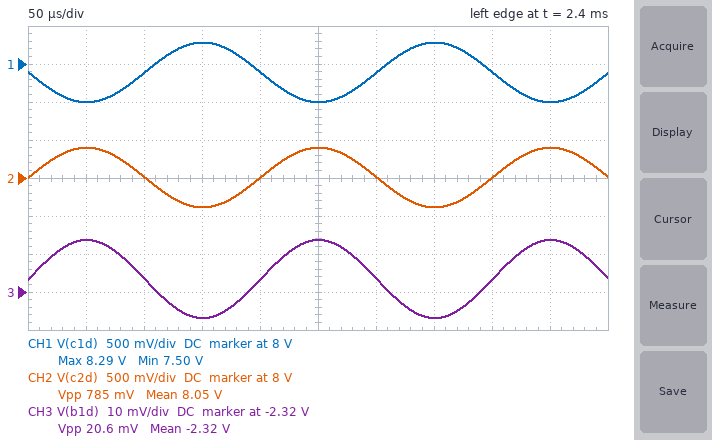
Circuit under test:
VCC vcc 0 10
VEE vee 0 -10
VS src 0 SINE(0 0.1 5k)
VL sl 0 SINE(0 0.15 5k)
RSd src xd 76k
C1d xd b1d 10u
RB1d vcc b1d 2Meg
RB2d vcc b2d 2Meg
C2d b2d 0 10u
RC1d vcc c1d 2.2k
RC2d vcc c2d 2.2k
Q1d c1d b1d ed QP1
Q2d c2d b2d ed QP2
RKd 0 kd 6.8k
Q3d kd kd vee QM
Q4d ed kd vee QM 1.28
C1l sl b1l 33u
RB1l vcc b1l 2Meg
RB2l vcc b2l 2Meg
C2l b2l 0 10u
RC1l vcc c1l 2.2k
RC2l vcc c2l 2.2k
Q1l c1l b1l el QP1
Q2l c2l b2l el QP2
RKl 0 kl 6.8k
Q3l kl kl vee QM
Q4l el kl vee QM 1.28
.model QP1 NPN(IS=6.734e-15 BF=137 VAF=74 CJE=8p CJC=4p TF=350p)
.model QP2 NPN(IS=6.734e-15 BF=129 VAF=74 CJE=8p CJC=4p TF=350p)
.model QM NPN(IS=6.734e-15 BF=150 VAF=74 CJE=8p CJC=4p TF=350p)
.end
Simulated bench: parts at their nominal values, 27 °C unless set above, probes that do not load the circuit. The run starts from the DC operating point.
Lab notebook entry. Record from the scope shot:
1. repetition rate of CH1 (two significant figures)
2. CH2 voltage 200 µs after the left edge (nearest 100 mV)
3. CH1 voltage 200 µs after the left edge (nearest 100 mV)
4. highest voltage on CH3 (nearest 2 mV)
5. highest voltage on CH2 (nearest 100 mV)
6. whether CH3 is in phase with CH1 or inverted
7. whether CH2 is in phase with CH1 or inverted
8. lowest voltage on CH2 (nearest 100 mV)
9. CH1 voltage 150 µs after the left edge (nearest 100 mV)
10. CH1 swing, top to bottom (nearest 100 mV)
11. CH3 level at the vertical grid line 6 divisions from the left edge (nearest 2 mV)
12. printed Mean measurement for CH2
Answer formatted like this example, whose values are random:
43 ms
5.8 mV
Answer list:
5.0 kHz
8.0 V
7.9 V
-2.306 V
8.4 V
inverted
inverted
7.6 V
8.3 V
800 mV
-2.316 V
8.05 V
